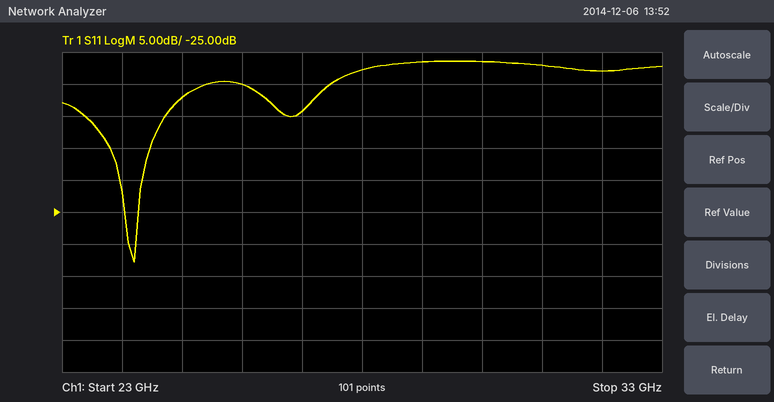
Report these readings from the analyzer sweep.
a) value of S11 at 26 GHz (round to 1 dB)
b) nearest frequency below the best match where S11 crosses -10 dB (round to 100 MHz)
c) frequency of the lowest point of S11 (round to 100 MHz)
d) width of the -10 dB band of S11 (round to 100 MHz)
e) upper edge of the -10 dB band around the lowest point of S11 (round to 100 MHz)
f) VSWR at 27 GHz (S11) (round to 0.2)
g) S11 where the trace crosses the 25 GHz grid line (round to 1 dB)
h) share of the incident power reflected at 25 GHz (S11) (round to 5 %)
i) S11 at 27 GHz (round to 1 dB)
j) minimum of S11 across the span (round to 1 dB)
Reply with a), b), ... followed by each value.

a) -5 dB
b) 23.4 GHz
c) 24.2 GHz
d) 1.3 GHz
e) 24.7 GHz
f) 2.0
g) -7 dB
h) 20 %
i) -9 dB
j) -33 dB
